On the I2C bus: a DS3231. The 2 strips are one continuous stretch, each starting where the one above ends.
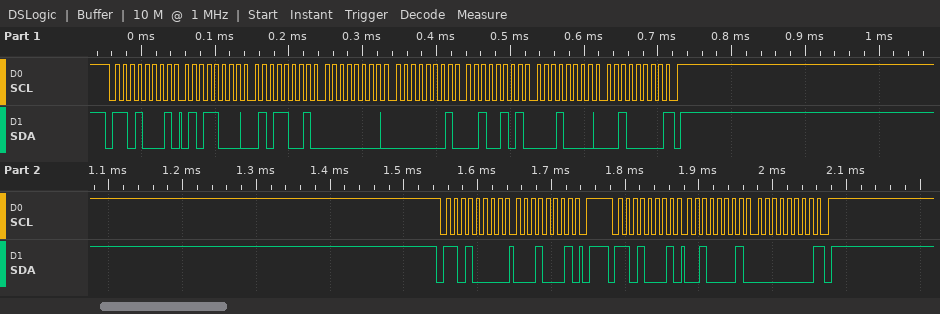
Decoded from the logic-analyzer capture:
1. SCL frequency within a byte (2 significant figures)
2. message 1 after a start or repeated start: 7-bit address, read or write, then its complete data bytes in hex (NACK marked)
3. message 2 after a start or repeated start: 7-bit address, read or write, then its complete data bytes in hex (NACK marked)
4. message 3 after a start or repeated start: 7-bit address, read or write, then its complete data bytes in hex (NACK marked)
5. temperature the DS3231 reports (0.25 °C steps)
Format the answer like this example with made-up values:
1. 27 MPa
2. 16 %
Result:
1. 100 kHz
2. 0x68 read: 58 59 00 01 25 10 20 NACK
3. 0x68 write: 11
4. 0x68 read: 21 00 NACK
5. 33.00 °C
